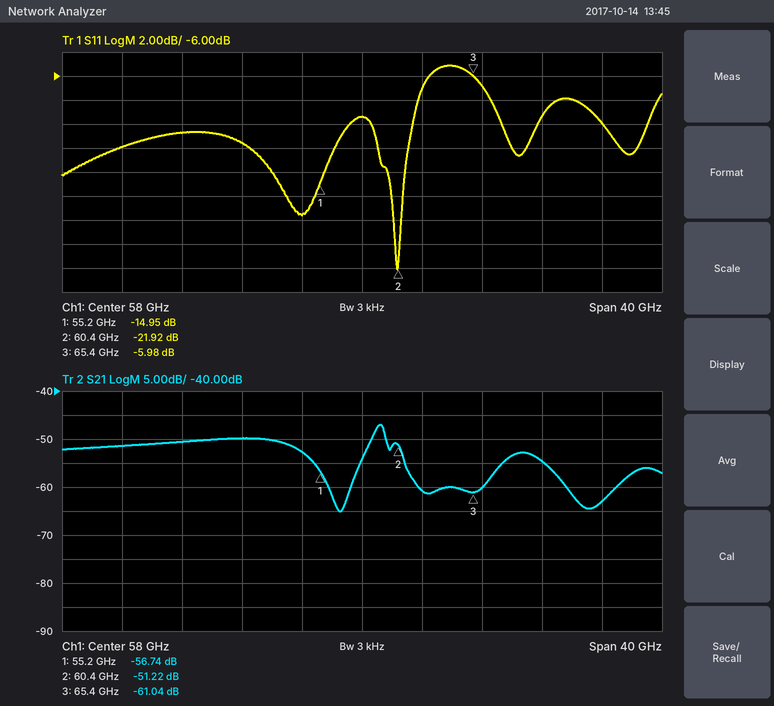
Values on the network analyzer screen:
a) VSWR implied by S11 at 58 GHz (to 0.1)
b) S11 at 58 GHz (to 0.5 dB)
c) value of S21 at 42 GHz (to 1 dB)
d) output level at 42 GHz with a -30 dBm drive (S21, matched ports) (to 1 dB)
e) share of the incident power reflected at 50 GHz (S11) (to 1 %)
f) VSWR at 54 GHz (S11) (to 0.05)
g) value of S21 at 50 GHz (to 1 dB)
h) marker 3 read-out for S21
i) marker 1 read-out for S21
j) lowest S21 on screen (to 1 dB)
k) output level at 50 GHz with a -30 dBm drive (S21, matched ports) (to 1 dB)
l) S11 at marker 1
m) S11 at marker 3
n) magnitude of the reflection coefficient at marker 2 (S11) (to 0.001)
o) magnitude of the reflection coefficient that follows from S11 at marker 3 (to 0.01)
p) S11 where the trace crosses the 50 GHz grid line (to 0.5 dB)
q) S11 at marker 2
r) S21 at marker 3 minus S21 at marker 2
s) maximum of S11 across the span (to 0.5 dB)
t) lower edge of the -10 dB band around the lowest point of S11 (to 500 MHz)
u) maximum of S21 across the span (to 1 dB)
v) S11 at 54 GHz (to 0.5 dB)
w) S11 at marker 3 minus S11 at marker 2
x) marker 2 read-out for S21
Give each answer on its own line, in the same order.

2.0
-9.5 dB
-51 dB
-81 dBm
7 %
1.30
-50 dB
-61.04 dB
-56.74 dB
-65 dB
-80 dBm
-14.95 dB
-5.98 dB
0.080
0.50
-11.5 dB
-21.92 dB
-9.82 dB
-5.0 dB
58.5 GHz
-47 dB
-17.5 dB
15.94 dB
-51.22 dB
